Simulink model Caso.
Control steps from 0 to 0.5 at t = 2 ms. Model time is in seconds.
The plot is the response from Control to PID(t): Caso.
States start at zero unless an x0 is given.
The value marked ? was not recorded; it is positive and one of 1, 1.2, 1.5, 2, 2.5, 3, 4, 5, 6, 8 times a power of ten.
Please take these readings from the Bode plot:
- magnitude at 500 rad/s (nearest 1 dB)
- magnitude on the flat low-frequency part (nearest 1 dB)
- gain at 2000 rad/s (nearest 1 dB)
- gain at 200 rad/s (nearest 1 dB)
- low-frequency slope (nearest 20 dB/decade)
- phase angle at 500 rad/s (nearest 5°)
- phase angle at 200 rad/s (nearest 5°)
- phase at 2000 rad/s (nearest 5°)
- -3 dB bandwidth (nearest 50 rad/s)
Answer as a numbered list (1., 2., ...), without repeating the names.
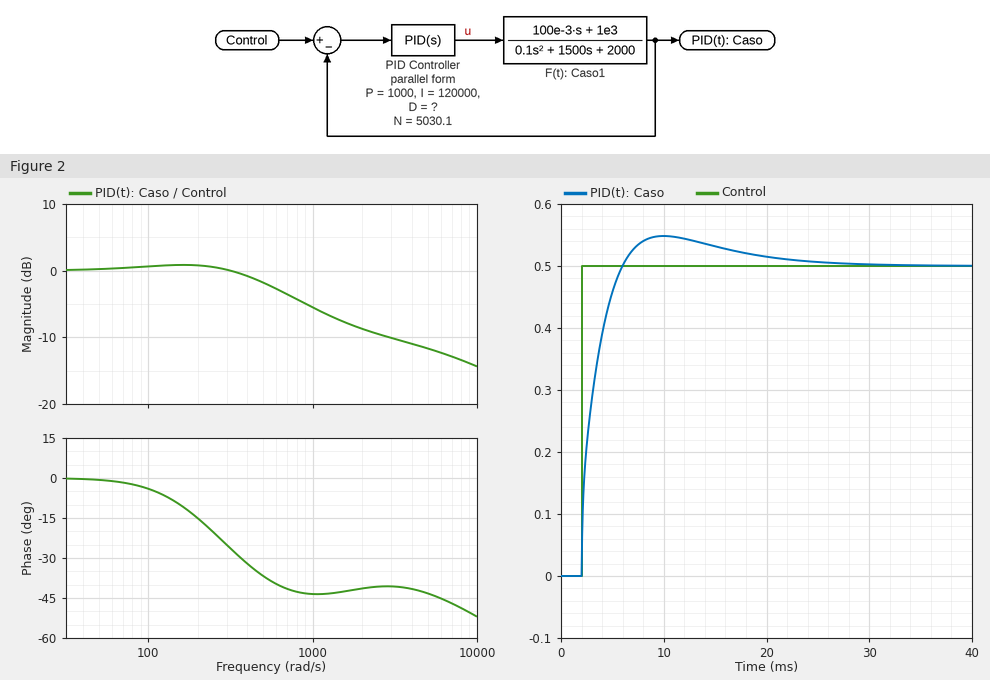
1. -2 dB
2. 0 dB
3. -9 dB
4. 1 dB
5. 0 dB/decade
6. -35°
7. -15°
8. -40°
9. 600 rad/s
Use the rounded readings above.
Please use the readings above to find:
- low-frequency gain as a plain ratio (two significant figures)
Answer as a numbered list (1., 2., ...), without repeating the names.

1. 1.0
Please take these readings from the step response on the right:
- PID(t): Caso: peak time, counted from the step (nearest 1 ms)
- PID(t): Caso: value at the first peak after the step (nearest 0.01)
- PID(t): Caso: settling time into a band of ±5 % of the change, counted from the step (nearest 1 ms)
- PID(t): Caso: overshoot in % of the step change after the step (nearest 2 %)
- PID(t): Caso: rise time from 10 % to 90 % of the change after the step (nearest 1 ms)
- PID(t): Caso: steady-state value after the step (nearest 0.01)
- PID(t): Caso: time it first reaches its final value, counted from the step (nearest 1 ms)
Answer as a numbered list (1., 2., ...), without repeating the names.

1. 8 ms
2. 0.55
3. 15 ms
4. 10 %
5. 3 ms
6. 0.50
7. 4 ms
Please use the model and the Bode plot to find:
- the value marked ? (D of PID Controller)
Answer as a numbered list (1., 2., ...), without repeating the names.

1. 0.4
